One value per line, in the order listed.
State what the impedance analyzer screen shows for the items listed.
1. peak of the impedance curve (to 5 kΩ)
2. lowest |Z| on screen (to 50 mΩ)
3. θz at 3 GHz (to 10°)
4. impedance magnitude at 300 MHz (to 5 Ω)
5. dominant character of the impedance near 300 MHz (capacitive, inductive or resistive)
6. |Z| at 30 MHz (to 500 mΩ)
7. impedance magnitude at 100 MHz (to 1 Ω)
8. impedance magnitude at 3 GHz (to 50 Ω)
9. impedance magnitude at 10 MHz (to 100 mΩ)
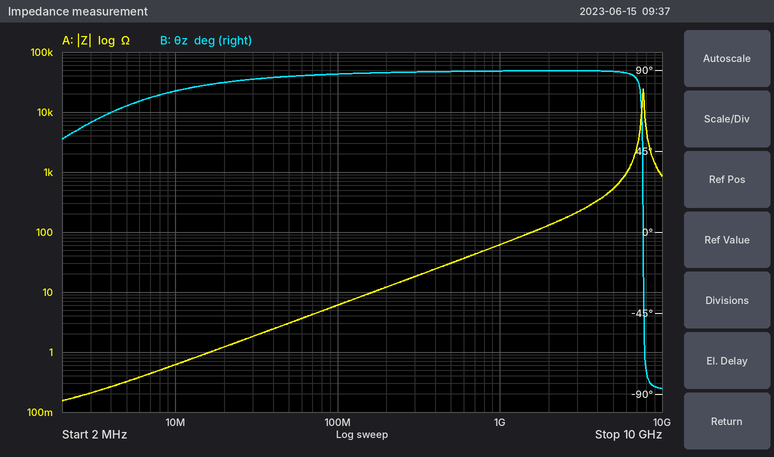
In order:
25 kΩ
150 mΩ
90°
20 Ω
inductive
2.0 Ω
6 Ω
200 Ω
600 mΩ
